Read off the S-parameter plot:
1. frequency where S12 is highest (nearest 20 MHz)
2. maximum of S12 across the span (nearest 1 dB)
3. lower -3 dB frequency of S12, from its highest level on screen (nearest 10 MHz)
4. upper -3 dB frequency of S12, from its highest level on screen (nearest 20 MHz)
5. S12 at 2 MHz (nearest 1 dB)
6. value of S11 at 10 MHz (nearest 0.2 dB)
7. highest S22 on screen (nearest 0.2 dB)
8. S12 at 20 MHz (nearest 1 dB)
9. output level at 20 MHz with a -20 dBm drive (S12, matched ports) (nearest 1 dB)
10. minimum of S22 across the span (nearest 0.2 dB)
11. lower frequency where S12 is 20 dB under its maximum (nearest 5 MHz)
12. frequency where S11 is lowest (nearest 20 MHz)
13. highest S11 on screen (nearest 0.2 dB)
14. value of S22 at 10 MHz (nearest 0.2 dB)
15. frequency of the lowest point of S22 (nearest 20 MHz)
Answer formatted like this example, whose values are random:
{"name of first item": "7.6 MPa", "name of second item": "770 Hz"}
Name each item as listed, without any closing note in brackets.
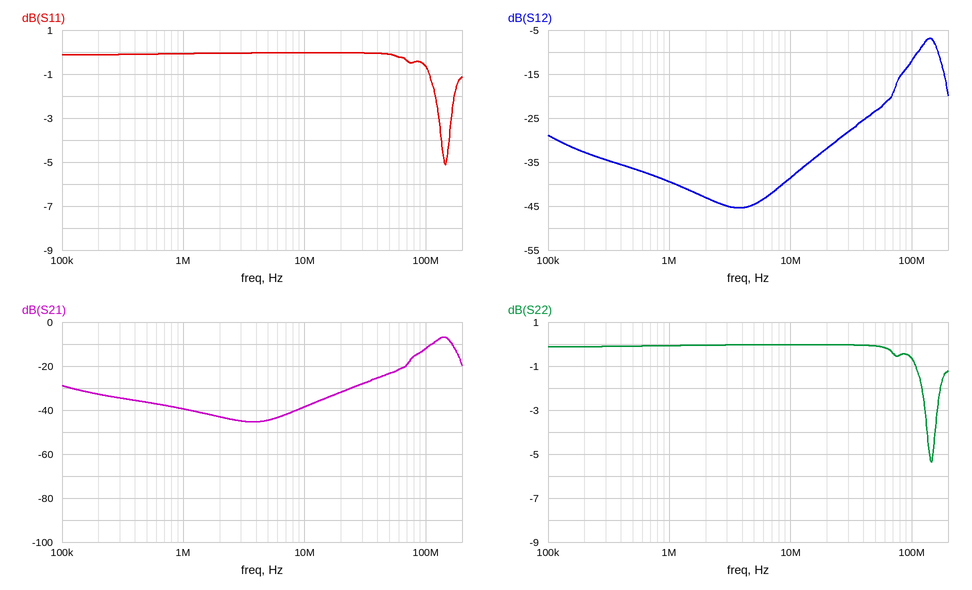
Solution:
{"frequency where S12 is highest": "140 MHz", "maximum of S12 across the span": "-7 dB", "lower -3 dB frequency of S12, from its highest level on screen": "110 MHz", "upper -3 dB frequency of S12, from its highest level on screen": "160 MHz", "S12 at 2 MHz": "-43 dB", "value of S11 at 10 MHz": "0.0 dB", "highest S22 on screen": "0.0 dB", "S12 at 20 MHz": "-32 dB", "output level at 20 MHz with a -20 dBm drive (S12, matched ports)": "-52 dBm", "minimum of S22 across the span": "-5.4 dB", "lower frequency where S12 is 20 dB under its maximum": "35 MHz", "frequency where S11 is lowest": "140 MHz", "highest S11 on screen": "0.0 dB", "value of S22 at 10 MHz": "0.0 dB", "frequency of the lowest point of S22": "140 MHz"}
